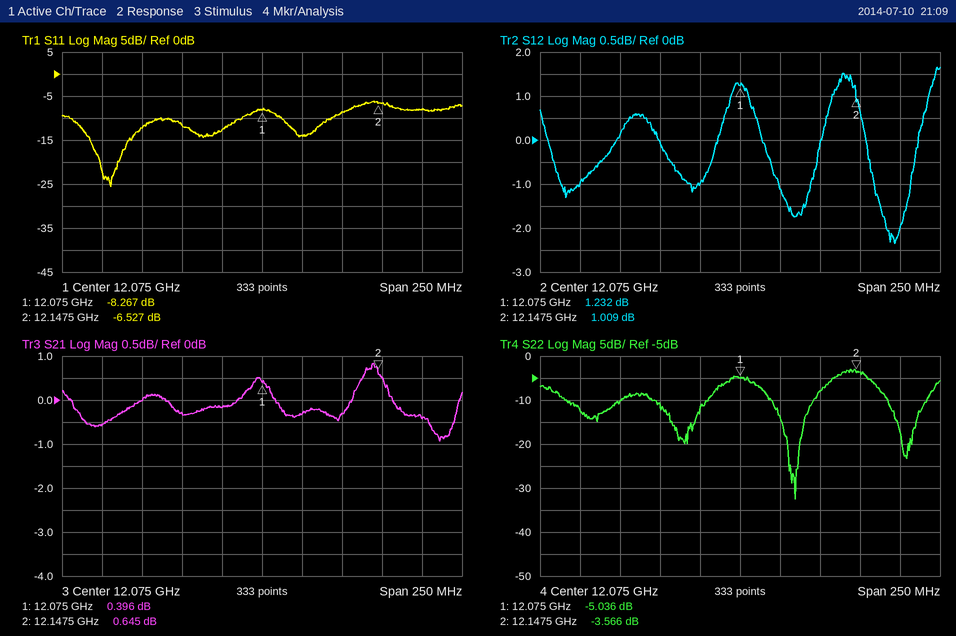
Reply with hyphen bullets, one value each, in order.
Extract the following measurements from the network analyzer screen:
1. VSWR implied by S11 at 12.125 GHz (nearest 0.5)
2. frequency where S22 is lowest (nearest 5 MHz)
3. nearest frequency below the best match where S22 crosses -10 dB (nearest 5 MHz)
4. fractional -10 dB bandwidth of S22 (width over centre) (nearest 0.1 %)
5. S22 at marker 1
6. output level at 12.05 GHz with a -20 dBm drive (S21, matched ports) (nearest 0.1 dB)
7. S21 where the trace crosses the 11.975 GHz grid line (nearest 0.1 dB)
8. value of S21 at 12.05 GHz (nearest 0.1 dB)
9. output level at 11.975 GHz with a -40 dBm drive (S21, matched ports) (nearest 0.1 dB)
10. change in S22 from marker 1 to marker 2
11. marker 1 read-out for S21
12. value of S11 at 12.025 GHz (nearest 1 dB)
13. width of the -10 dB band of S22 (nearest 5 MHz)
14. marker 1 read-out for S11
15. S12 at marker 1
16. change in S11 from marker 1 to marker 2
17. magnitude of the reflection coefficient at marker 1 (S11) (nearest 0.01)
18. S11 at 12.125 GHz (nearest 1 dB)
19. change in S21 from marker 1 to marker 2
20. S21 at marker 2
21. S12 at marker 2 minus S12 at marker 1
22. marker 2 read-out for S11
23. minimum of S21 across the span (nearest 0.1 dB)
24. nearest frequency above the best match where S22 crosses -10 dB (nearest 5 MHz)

- 2.0
- 12.110 GHz
- 12.095 GHz
- 0.2 %
- -5.036 dB
- -20.2 dBm
- -0.6 dB
- -0.2 dB
- -40.6 dBm
- 1.470 dB
- 0.396 dB
- -12 dB
- 25 MHz
- -8.267 dB
- 1.232 dB
- 1.740 dB
- 0.39
- -9 dB
- 0.249 dB
- 0.645 dB
- -0.223 dB
- -6.527 dB
- -0.9 dB
- 12.120 GHz
